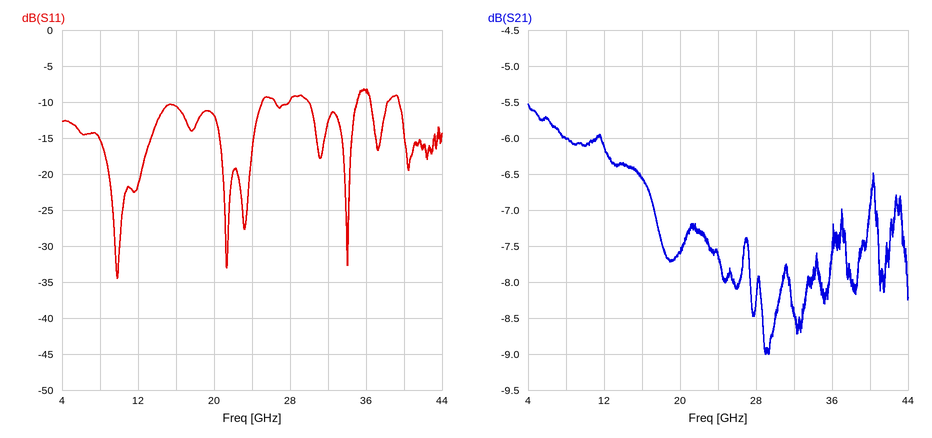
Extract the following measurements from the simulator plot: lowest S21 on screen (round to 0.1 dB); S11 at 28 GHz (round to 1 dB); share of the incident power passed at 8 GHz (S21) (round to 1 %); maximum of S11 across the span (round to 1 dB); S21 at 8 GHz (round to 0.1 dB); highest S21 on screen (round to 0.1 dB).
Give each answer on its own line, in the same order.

-9.0 dB
-10 dB
25 %
-8 dB
-6.0 dB
-5.5 dB
